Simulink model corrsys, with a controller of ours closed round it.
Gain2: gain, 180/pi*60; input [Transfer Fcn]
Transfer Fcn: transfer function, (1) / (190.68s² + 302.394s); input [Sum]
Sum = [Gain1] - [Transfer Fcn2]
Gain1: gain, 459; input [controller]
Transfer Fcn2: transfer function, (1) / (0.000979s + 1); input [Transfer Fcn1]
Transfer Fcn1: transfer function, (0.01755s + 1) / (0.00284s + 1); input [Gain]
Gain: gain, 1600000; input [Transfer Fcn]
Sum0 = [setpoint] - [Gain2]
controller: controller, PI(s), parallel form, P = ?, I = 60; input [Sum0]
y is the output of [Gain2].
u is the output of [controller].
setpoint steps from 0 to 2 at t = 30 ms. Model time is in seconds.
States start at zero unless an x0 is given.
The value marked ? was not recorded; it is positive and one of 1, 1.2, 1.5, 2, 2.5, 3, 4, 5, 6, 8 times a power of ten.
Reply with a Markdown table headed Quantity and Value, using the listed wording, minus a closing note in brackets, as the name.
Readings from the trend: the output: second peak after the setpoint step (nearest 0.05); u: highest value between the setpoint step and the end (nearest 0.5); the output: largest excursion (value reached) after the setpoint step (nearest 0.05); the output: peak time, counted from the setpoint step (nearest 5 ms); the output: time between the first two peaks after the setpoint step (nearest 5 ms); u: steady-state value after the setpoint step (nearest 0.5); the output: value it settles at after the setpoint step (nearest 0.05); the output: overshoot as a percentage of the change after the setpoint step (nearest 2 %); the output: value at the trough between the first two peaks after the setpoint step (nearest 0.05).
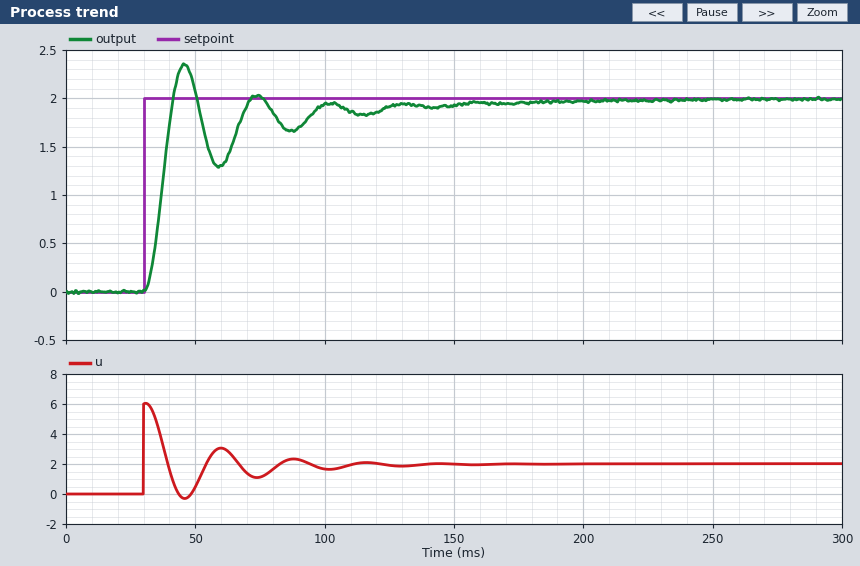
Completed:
| Quantity | Value |
|---|---|
| the output: second peak after the setpoint step | 2.05 |
| u: highest value between the setpoint step and the end | 6.0 |
| the output: largest excursion (value reached) after the setpoint step | 2.35 |
| the output: peak time, counted from the setpoint step | 15 ms |
| the output: time between the first two peaks after the setpoint step | 30 ms |
| u: steady-state value after the setpoint step | 2.0 |
| the output: value it settles at after the setpoint step | 2.00 |
| the output: overshoot as a percentage of the change after the setpoint step | 18 % |
| the output: value at the trough between the first two peaks after the setpoint step | 1.30 |
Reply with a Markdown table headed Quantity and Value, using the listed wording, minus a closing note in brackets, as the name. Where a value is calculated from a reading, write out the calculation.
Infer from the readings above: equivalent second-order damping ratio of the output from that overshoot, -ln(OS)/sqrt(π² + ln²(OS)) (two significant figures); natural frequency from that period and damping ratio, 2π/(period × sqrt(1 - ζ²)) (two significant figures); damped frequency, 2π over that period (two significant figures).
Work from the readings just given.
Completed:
| Quantity | Value |
|---|---|
| equivalent second-order damping ratio of the output from that overshoot, -ln(OS)/sqrt(π² + ln²(OS)) | ln(0.18) = -1.715; 1.715 / sqrt(9.870 + 2.941) = 0.48 |
| natural frequency from that period and damping ratio, 2π/(period × sqrt(1 - ζ²)) | 2π / (30 × sqrt(1 - 0.48²)) = 0.24 rad/ms |
| damped frequency, 2π over that period | 2π / 30 = 0.21 rad/ms |
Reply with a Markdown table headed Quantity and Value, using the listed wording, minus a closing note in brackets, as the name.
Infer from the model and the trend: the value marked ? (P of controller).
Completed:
| Quantity | Value |
|---|---|
| the value marked ? | 3 |
